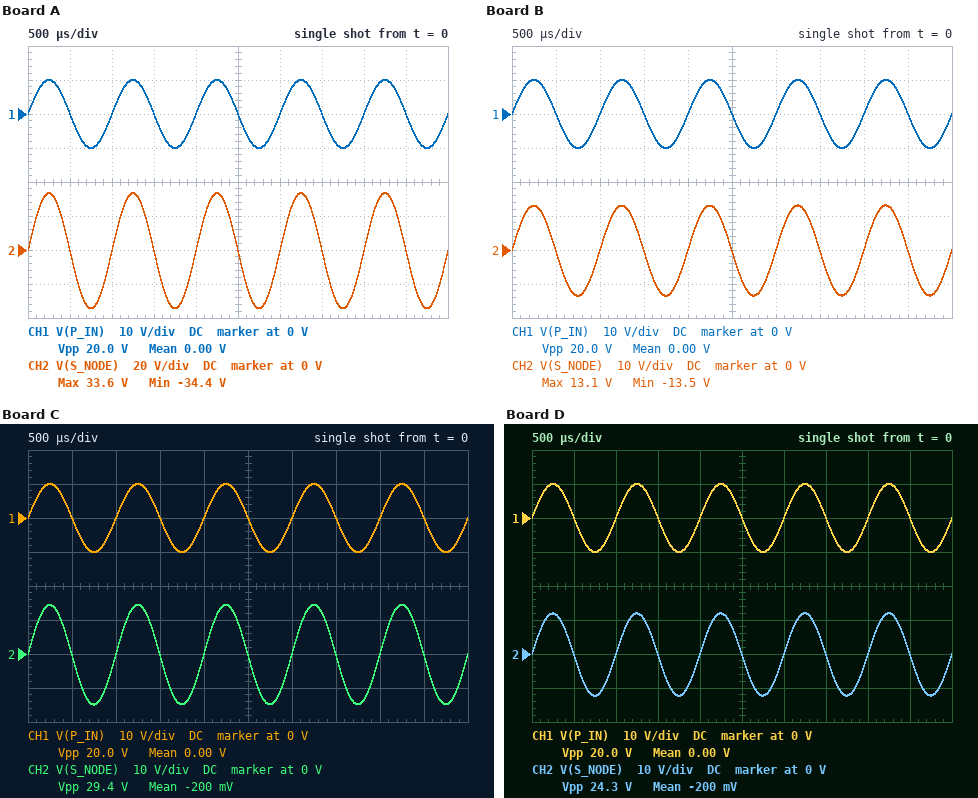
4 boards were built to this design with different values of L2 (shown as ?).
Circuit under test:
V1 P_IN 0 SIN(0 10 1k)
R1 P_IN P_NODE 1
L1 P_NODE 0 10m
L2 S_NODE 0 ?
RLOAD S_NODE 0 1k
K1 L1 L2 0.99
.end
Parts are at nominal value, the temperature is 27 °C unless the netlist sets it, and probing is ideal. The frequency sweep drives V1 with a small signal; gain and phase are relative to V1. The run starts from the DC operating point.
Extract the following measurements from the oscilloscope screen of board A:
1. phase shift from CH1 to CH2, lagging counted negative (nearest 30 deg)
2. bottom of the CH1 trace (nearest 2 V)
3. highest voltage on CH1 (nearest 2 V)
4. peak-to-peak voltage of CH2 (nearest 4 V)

0 deg
-10 V
10 V
68 V
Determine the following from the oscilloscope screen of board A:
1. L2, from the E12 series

120 mH
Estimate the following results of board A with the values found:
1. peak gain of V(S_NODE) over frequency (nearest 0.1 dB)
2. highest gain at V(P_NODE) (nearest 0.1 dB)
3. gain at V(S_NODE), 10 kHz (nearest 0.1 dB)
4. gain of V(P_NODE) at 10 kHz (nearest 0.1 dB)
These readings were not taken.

10.6 dB
0 dB
10.5 dB
-0.1 dB
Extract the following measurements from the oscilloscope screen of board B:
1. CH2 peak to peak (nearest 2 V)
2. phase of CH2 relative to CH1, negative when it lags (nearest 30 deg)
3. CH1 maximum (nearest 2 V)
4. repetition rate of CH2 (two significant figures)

26 V
0 deg
10 V
1.0 kHz
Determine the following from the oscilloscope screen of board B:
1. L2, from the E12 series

18 mH
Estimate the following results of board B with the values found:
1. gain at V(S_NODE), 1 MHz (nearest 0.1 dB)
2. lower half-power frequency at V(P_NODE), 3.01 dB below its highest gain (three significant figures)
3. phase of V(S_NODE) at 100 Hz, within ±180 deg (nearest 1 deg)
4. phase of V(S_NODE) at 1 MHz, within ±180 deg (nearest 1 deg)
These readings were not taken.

-5.4 dB
15.9 Hz
9 deg
-66 deg
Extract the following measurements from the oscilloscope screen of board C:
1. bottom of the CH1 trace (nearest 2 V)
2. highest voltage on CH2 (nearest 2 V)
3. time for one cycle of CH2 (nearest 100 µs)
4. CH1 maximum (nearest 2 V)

-10 V
14 V
1.0 ms
10 V
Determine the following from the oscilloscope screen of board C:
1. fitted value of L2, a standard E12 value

22 mH
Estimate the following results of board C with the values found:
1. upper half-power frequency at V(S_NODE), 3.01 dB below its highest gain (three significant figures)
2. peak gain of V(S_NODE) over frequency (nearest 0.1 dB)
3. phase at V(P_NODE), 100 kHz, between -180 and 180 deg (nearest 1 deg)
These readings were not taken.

364 kHz
3.3 dB
0 deg
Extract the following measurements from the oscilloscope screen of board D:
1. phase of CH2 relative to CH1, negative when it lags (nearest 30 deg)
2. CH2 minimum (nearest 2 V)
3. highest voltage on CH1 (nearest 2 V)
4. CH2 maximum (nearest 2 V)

0 deg
-12 V
10 V
12 V
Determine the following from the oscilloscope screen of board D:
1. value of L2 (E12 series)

15 mH
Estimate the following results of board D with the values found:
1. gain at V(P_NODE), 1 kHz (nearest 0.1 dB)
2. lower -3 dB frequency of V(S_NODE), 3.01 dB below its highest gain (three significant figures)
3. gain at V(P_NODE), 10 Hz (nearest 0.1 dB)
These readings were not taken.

0 dB
15.9 Hz
-5.5 dB
